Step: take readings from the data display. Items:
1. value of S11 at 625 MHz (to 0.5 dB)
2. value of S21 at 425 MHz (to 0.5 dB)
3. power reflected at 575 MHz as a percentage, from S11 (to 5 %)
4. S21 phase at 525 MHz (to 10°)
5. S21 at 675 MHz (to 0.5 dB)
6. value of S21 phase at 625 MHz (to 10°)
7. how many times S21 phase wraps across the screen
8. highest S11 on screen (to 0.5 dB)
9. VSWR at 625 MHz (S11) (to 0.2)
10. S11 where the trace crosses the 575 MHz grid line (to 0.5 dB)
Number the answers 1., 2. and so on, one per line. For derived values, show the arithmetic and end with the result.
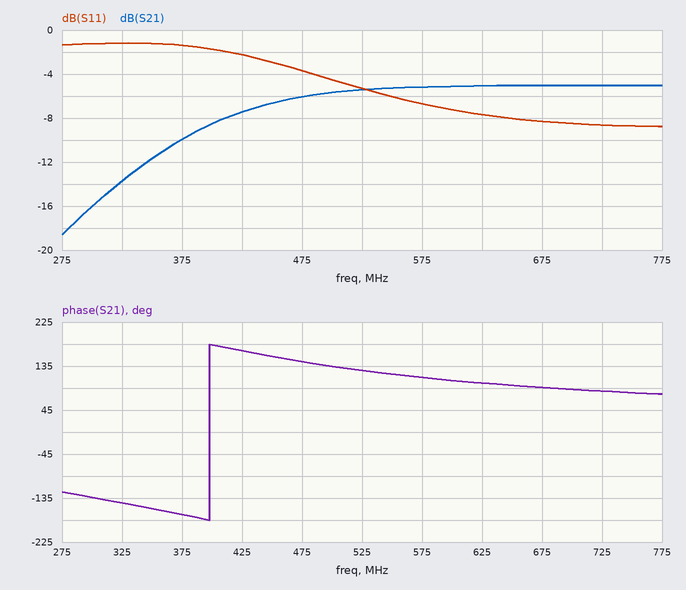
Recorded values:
1. -7.5 dB
2. -7.5 dB
3. 10^(-6.5/10) ≈ 22.4 %, so 20 % to the nearest 5 %
4. 130°
5. -5.0 dB
6. 100°
7. 1
8. -1.0 dB
9. |Γ| = 10^(-7.5/20) = 0.4217; VSWR = (1 + 0.4217)/(1 − 0.4217) ≈ 2.46, so 2.4 to the nearest 0.2
10. -6.5 dB
